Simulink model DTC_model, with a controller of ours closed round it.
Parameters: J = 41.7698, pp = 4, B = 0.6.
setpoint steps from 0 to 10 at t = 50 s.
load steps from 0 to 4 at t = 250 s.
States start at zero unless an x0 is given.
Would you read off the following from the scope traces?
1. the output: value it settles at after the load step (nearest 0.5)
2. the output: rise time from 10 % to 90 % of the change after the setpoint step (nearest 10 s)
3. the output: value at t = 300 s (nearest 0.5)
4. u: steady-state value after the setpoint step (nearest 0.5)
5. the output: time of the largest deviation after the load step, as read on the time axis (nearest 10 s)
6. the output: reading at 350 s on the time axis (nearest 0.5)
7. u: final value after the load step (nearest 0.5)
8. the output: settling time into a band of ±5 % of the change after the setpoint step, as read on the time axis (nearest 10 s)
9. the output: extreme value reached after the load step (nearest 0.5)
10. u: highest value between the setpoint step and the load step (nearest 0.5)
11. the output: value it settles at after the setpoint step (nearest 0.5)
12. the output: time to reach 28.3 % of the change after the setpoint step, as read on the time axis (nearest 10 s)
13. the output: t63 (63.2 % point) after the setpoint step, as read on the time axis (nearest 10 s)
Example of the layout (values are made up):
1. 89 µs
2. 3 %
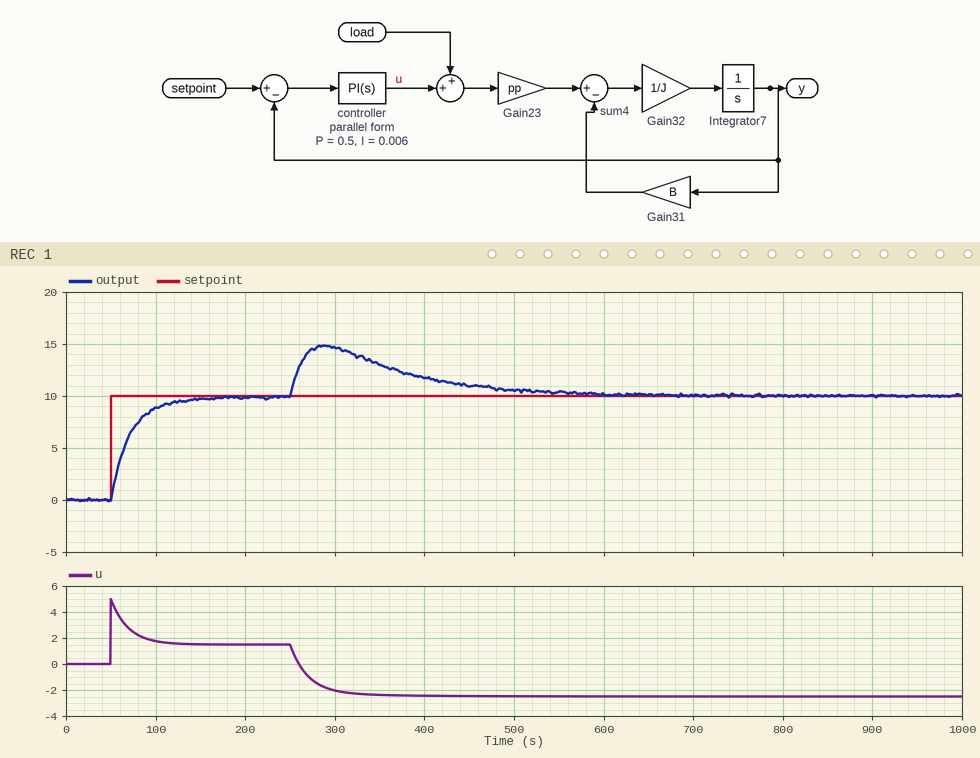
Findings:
1. 10.0
2. 50 s
3. 14.5
4. 1.5
5. 290 s
6. 13.0
7. -2.5
8. 130 s
9. 15.0
10. 5.0
11. 10.0
12. 60 s
13. 70 s
